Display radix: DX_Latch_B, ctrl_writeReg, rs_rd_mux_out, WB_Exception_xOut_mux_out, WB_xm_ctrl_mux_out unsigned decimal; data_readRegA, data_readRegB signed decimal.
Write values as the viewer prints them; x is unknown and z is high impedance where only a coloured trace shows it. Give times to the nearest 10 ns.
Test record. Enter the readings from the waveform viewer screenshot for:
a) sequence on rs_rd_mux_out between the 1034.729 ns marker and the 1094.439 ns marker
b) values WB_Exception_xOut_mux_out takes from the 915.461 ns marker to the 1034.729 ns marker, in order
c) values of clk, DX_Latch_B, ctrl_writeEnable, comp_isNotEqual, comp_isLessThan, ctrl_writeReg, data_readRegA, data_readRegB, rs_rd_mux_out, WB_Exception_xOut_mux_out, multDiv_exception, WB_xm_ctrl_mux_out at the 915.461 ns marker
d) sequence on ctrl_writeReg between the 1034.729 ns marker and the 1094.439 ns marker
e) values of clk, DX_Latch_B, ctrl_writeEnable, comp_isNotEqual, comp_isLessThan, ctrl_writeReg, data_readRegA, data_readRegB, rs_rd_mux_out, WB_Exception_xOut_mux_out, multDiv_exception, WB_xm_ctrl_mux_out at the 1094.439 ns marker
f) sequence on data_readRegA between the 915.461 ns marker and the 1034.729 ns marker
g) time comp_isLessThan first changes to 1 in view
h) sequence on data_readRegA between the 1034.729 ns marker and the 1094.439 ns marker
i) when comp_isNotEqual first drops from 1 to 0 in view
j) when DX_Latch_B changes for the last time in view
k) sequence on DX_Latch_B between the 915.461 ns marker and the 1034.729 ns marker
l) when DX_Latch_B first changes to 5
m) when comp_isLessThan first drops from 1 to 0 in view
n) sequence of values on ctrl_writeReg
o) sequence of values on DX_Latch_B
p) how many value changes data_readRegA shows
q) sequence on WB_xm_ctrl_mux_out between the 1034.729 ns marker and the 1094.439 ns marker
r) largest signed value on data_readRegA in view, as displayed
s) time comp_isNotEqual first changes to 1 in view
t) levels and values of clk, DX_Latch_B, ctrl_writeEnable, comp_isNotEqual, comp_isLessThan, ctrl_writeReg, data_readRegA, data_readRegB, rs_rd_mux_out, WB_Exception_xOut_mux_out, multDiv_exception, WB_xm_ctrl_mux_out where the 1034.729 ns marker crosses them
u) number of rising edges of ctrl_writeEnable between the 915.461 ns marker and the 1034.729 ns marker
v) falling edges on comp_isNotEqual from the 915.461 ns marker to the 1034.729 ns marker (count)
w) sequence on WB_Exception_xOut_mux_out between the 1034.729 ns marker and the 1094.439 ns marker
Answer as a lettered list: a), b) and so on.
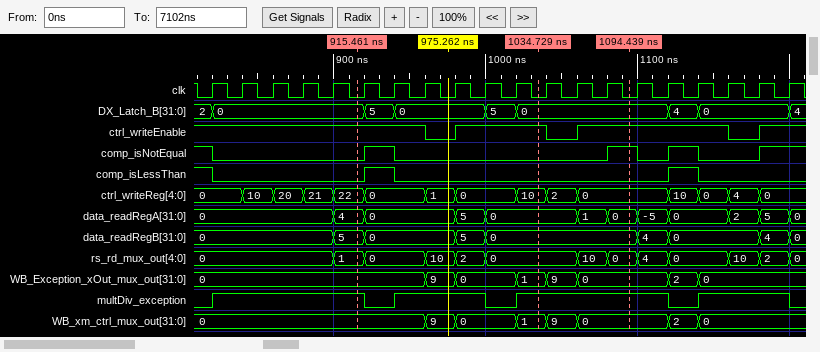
a) 0, 10, 0
b) 0, 9, 0, 1
c) clk=0, DX_Latch_B=0, ctrl_writeEnable=1, comp_isNotEqual=0, comp_isLessThan=0, ctrl_writeReg=22, data_readRegA=4, data_readRegB=5, rs_rd_mux_out=1, WB_Exception_xOut_mux_out=0, multDiv_exception=1, WB_xm_ctrl_mux_out=0
d) 10, 2, 0
e) clk=0, DX_Latch_B=0, ctrl_writeEnable=1, comp_isNotEqual=1, comp_isLessThan=0, ctrl_writeReg=0, data_readRegA=0, data_readRegB=0, rs_rd_mux_out=0, WB_Exception_xOut_mux_out=0, multDiv_exception=1, WB_xm_ctrl_mux_out=0
f) 4, 0, 5, 0
g) 920 ns
h) 0, 1, 0
i) 820 ns
j) 1200 ns
k) 0, 5, 0, 5, 0
l) 920 ns
m) 820 ns
n) 0, 10, 20, 21, 22, 0, 1, 0, 10, 2, 0, 10, 0, 4, 0
o) 2, 0, 5, 0, 5, 0, 4, 0, 4
p) 11
q) 1, 9, 0
r) 5
s) 920 ns
t) clk=0, DX_Latch_B=0, ctrl_writeEnable=1, comp_isNotEqual=0, comp_isLessThan=0, ctrl_writeReg=10, data_readRegA=0, data_readRegB=0, rs_rd_mux_out=0, WB_Exception_xOut_mux_out=1, multDiv_exception=1, WB_xm_ctrl_mux_out=1
u) 1
v) 1
w) 1, 9, 0
